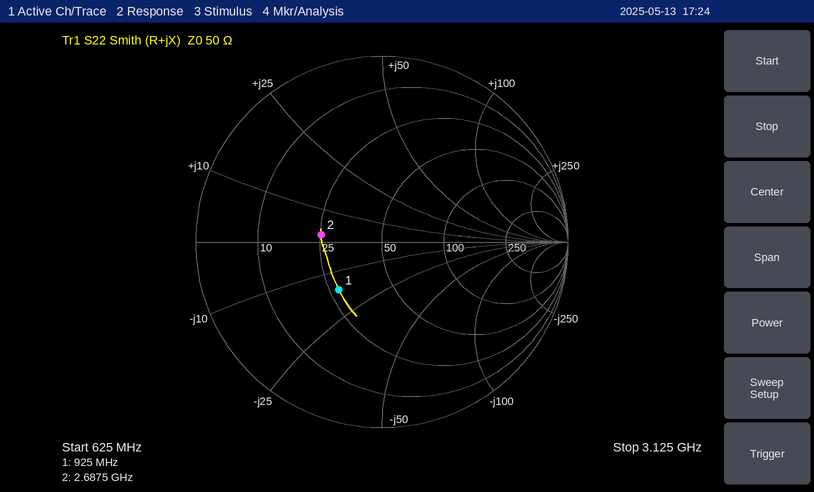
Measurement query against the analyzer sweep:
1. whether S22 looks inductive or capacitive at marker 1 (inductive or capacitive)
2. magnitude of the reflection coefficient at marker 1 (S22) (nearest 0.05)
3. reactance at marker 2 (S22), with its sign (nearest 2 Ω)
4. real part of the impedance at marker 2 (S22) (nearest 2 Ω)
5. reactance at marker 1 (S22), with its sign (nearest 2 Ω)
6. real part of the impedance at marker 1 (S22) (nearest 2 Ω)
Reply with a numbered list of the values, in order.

1. capacitive
2. 0.35
3. +2 Ω
4. 26 Ω
5. -16 Ω
6. 28 Ω
